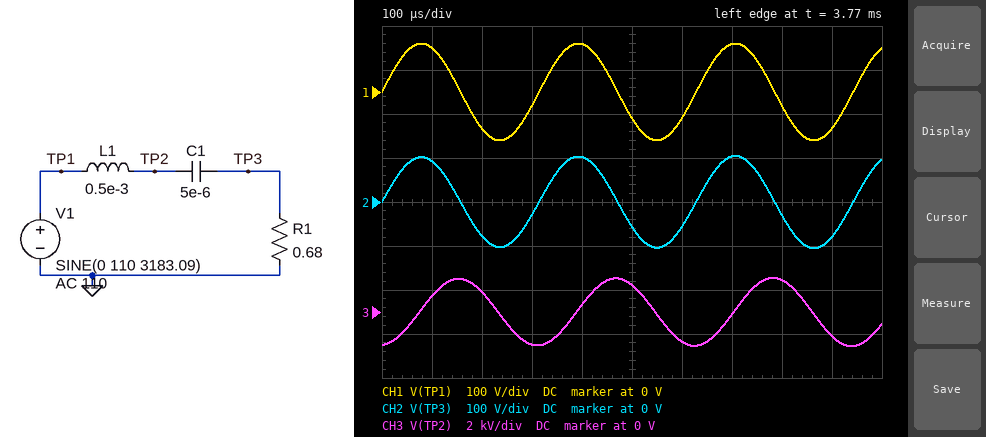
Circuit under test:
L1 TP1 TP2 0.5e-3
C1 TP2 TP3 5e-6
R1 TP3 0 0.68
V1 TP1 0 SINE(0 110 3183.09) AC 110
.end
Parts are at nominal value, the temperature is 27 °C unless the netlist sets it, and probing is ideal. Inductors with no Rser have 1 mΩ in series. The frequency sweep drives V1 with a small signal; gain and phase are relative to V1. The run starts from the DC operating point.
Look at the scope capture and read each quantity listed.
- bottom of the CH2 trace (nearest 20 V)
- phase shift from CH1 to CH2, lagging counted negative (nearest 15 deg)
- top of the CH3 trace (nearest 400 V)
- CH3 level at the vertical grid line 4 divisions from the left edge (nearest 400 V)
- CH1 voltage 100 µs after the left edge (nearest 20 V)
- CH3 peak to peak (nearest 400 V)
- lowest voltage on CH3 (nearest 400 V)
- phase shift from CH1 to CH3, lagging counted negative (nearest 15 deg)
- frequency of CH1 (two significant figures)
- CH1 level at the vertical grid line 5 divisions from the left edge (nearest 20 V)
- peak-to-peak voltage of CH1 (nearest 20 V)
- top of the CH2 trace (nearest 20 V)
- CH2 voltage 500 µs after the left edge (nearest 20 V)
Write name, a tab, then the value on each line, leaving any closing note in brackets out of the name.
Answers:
bottom of the CH2 trace	-100 V
phase shift from CH1 to CH2, lagging counted negative	0 deg
top of the CH3 trace	1.6 kV
CH3 level at the vertical grid line 4 divisions from the left edge	400 V
CH1 voltage 100 µs after the left edge	100 V
CH3 peak to peak	3.2 kV
lowest voltage on CH3	-1.6 kV
phase shift from CH1 to CH3, lagging counted negative	-90 deg
frequency of CH1	3.2 kHz
CH1 level at the vertical grid line 5 divisions from the left edge	-60 V
peak-to-peak voltage of CH1	220 V
top of the CH2 trace	100 V
CH2 voltage 500 µs after the left edge	-60 V
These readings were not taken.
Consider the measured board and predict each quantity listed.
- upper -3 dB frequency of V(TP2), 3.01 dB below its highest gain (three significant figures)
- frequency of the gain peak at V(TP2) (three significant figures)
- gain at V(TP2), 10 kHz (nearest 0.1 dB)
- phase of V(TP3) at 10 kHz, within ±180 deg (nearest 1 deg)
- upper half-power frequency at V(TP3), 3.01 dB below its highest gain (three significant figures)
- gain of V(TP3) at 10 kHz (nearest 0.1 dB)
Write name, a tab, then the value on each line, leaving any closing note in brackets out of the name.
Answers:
upper -3 dB frequency of V(TP2), 3.01 dB below its highest gain	3.29 kHz
frequency of the gain peak at V(TP2)	3.18 kHz
gain at V(TP2), 10 kHz	-18.8 dB
phase of V(TP3) at 10 kHz, within ±180 deg	-89 deg
upper half-power frequency at V(TP3), 3.01 dB below its highest gain	3.29 kHz
gain of V(TP3) at 10 kHz	-32.4 dB
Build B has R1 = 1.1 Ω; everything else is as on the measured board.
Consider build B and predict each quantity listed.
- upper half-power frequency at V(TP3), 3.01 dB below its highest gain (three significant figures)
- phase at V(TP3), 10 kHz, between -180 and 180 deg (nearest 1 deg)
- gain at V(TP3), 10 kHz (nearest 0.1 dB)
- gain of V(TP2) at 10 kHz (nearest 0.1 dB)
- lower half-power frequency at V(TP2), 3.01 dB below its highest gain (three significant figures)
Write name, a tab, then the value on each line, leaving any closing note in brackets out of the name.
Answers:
upper half-power frequency at V(TP3), 3.01 dB below its highest gain	3.36 kHz
phase at V(TP3), 10 kHz, between -180 and 180 deg	-88 deg
gain at V(TP3), 10 kHz	-28.2 dB
gain of V(TP2) at 10 kHz	-18.5 dB
lower half-power frequency at V(TP2), 3.01 dB below its highest gain	2.99 kHz
